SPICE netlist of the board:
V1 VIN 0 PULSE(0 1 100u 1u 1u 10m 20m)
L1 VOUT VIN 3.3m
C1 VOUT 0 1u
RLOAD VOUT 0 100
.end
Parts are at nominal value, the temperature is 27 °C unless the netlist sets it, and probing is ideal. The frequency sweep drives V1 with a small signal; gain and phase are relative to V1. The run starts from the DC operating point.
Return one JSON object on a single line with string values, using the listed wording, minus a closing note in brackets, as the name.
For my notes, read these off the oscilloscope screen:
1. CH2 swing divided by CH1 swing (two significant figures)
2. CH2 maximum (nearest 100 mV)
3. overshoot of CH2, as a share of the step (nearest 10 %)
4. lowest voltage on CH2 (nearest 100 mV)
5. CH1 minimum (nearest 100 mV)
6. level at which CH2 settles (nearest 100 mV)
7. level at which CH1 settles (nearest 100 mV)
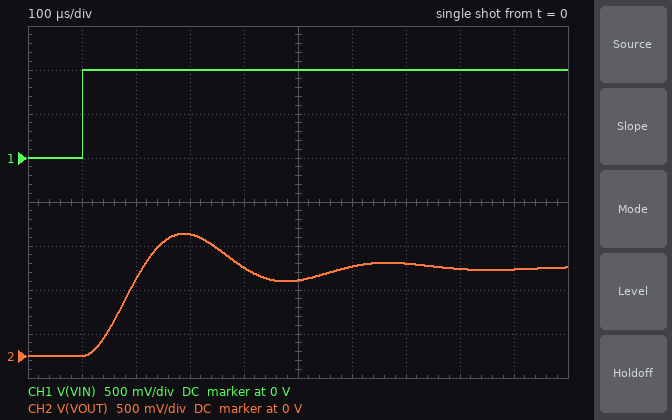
{"CH2 swing divided by CH1 swing": "1.4", "CH2 maximum": "1.4 V", "overshoot of CH2, as a share of the step": "40 %", "lowest voltage on CH2": "0 V", "CH1 minimum": "0 V", "level at which CH2 settles": "1.0 V", "level at which CH1 settles": "1.0 V"}
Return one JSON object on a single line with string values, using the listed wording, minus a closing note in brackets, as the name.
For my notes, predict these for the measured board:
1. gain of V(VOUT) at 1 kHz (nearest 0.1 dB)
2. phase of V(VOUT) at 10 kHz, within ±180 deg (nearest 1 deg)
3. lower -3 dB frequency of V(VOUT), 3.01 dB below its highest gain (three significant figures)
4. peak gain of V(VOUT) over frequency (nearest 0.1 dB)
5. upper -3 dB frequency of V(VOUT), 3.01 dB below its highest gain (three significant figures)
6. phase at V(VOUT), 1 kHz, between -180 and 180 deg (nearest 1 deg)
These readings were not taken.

{"gain of V(VOUT) at 1 kHz": "1.0 dB", "phase of V(VOUT) at 10 kHz, within ±180 deg": "-170 deg", "lower -3 dB frequency of V(VOUT), 3.01 dB below its highest gain": "1.48 kHz", "peak gain of V(VOUT) over frequency": "5.2 dB", "upper -3 dB frequency of V(VOUT), 3.01 dB below its highest gain": "3.26 kHz", "phase at V(VOUT), 1 kHz, between -180 and 180 deg": "-13 deg"}
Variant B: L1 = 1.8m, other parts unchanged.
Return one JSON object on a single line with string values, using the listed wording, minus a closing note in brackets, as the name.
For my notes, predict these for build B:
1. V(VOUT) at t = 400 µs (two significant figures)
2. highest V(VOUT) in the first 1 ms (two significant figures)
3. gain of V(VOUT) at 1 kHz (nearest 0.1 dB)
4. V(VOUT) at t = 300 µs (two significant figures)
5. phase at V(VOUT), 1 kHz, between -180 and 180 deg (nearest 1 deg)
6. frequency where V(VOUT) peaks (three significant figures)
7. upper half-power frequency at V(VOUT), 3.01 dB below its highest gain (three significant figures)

{"V(VOUT) at t = 400 µs": "790 mV", "highest V(VOUT) in the first 1 ms": "1.5 V", "gain of V(VOUT) at 1 kHz": "0.6 dB", "V(VOUT) at t = 300 µs": "1.1 V", "phase at V(VOUT), 1 kHz, between -180 and 180 deg": "-7 deg", "frequency where V(VOUT) peaks": "3.58 kHz", "upper half-power frequency at V(VOUT), 3.01 dB below its highest gain": "4.32 kHz"}
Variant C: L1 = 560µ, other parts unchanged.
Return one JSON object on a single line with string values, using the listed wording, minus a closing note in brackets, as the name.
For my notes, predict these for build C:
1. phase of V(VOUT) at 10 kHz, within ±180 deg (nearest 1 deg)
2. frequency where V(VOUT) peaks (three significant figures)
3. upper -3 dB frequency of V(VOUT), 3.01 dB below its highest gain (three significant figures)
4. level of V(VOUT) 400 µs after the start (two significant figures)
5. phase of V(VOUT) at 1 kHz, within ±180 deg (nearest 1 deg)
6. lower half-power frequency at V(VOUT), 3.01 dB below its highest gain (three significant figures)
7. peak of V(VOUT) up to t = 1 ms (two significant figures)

{"phase of V(VOUT) at 10 kHz, within ±180 deg": "-164 deg", "frequency where V(VOUT) peaks": "6.63 kHz", "upper -3 dB frequency of V(VOUT), 3.01 dB below its highest gain": "7.39 kHz", "level of V(VOUT) 400 µs after the start": "780 mV", "phase of V(VOUT) at 1 kHz, within ±180 deg": "-2 deg", "lower half-power frequency at V(VOUT), 3.01 dB below its highest gain": "5.77 kHz", "peak of V(VOUT) up to t = 1 ms": "1.7 V"}
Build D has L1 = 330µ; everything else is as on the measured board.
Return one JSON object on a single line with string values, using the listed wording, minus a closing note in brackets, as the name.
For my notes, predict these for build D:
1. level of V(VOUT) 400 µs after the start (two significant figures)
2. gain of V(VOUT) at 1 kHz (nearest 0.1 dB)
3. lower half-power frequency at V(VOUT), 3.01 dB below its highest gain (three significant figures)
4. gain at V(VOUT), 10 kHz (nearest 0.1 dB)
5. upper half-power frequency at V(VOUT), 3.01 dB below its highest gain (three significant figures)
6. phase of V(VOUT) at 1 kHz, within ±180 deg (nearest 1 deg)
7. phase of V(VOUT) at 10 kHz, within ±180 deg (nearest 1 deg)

{"level of V(VOUT) 400 µs after the start": "1.2 V", "gain of V(VOUT) at 1 kHz": "0.1 dB", "lower half-power frequency at V(VOUT), 3.01 dB below its highest gain": "7.85 kHz", "gain at V(VOUT), 10 kHz": "8.7 dB", "upper half-power frequency at V(VOUT), 3.01 dB below its highest gain": "9.45 kHz", "phase of V(VOUT) at 1 kHz, within ±180 deg": "-1 deg", "phase of V(VOUT) at 10 kHz, within ±180 deg": "-146 deg"}
